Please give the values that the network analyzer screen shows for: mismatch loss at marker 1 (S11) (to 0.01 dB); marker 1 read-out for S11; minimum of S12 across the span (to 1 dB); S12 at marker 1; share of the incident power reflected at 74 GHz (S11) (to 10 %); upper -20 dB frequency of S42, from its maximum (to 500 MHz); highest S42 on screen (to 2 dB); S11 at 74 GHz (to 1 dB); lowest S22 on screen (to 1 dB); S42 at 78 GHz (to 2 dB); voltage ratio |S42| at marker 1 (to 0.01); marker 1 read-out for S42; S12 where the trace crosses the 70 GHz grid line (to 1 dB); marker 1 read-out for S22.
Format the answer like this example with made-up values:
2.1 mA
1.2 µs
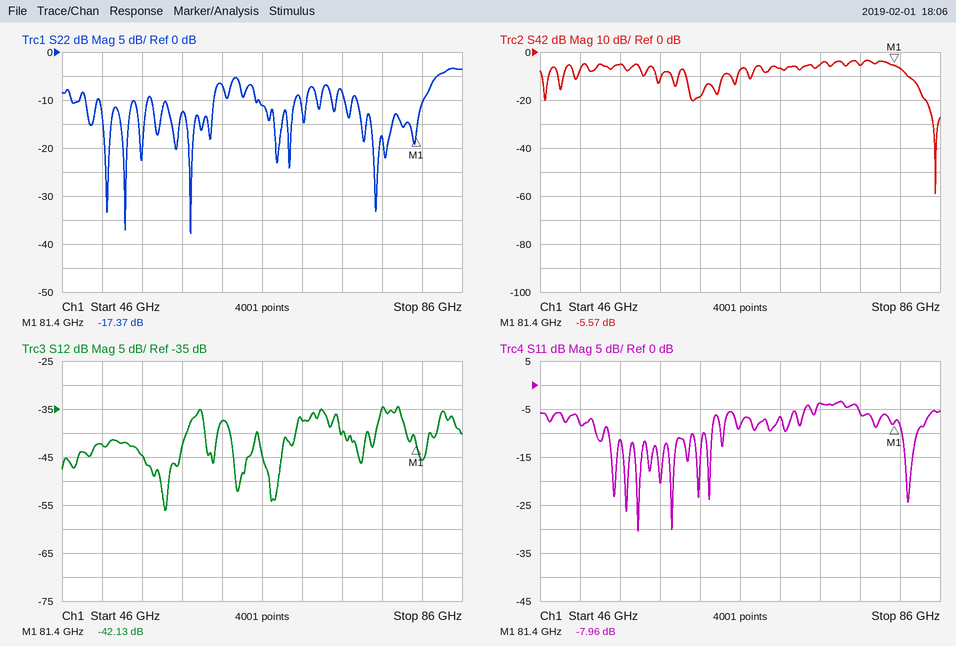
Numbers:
0.76 dB
-7.96 dB
-56 dB
-42.13 dB
40 %
85.0 GHz
-4 dB
-4 dB
-38 dB
-6 dB
0.53
-5.57 dB
-37 dB
-17.37 dB
